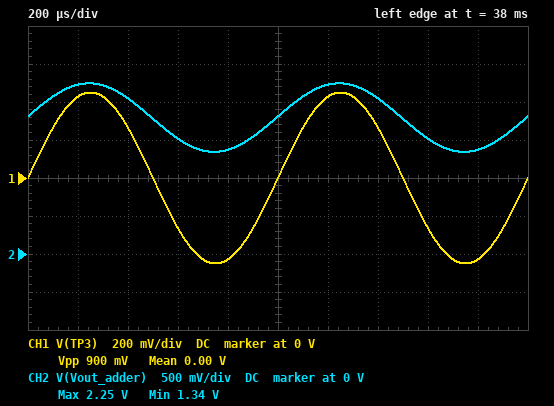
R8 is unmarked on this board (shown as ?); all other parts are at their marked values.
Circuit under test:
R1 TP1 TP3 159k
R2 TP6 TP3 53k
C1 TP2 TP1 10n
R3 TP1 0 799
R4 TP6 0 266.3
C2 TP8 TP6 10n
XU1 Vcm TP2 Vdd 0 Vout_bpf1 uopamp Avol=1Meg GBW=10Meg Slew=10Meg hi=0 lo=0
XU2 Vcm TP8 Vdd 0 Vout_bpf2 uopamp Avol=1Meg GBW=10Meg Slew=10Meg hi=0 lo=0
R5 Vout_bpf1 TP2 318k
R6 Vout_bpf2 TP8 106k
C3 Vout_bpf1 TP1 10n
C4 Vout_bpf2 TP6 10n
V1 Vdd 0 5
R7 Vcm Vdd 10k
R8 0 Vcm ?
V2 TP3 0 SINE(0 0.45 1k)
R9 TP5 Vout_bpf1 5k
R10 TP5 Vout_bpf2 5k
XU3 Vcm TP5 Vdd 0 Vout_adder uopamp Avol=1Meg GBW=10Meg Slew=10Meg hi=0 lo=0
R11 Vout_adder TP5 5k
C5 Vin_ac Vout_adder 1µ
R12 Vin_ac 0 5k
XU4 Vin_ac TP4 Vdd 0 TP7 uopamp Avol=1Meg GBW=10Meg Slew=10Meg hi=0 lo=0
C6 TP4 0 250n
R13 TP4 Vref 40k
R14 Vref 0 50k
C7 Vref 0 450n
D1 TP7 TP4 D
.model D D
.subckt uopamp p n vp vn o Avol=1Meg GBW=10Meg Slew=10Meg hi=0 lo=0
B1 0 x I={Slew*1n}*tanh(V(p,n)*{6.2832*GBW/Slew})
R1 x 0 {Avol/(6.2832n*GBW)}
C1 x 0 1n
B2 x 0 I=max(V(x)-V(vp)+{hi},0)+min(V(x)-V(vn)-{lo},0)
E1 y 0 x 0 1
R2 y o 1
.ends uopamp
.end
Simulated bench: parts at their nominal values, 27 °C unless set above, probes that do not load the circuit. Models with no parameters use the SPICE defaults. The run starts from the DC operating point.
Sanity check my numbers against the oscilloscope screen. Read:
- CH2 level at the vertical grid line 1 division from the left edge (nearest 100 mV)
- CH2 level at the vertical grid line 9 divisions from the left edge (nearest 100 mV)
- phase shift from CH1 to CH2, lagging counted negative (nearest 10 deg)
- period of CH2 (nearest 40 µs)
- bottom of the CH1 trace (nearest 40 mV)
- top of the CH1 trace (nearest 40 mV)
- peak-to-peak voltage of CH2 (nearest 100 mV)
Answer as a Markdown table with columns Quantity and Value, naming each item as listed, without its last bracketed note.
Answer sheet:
| Quantity | Value |
|---|---|
| CH2 level at the vertical grid line 1 division from the left edge | 2.2 V |
| CH2 level at the vertical grid line 9 divisions from the left edge | 1.4 V |
| phase shift from CH1 to CH2, lagging counted negative | 0 deg |
| period of CH2 | 1.00 ms |
| bottom of the CH1 trace | -440 mV |
| top of the CH1 trace | 440 mV |
| peak-to-peak voltage of CH2 | 900 mV |
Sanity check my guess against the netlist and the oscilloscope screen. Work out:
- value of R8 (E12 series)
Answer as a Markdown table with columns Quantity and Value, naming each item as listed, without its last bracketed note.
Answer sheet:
| Quantity | Value |
|---|---|
| value of R8 | 5.6 kΩ |
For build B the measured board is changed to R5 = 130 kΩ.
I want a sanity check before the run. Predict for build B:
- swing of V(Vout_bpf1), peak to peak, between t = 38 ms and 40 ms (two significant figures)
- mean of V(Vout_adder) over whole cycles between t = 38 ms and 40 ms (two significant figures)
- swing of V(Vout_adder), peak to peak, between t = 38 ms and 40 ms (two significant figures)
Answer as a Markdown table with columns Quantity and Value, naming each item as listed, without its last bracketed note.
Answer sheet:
| Quantity | Value |
|---|---|
| swing of V(Vout_bpf1), peak to peak, between t = 38 ms and 40 ms | 61 mV |
| mean of V(Vout_adder) over whole cycles between t = 38 ms and 40 ms | 1.8 V |
| swing of V(Vout_adder), peak to peak, between t = 38 ms and 40 ms | 95 mV |
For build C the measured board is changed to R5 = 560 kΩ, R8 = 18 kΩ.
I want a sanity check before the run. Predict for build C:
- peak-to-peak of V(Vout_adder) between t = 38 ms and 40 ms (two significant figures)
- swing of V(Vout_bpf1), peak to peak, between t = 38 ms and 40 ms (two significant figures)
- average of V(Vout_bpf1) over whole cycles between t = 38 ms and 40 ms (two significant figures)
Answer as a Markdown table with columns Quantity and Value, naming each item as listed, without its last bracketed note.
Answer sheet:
| Quantity | Value |
|---|---|
| peak-to-peak of V(Vout_adder) between t = 38 ms and 40 ms | 170 mV |
| swing of V(Vout_bpf1), peak to peak, between t = 38 ms and 40 ms | 210 mV |
| average of V(Vout_bpf1) over whole cycles between t = 38 ms and 40 ms | 3.2 V |
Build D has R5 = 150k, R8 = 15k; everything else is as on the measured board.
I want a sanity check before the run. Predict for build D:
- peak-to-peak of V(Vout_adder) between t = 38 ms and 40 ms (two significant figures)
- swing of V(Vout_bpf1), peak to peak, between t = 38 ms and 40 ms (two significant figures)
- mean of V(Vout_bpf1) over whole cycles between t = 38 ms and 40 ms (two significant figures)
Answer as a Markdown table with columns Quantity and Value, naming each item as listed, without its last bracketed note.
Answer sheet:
| Quantity | Value |
|---|---|
| peak-to-peak of V(Vout_adder) between t = 38 ms and 40 ms | 110 mV |
| swing of V(Vout_bpf1), peak to peak, between t = 38 ms and 40 ms | 79 mV |
| mean of V(Vout_bpf1) over whole cycles between t = 38 ms and 40 ms | 3.0 V |
